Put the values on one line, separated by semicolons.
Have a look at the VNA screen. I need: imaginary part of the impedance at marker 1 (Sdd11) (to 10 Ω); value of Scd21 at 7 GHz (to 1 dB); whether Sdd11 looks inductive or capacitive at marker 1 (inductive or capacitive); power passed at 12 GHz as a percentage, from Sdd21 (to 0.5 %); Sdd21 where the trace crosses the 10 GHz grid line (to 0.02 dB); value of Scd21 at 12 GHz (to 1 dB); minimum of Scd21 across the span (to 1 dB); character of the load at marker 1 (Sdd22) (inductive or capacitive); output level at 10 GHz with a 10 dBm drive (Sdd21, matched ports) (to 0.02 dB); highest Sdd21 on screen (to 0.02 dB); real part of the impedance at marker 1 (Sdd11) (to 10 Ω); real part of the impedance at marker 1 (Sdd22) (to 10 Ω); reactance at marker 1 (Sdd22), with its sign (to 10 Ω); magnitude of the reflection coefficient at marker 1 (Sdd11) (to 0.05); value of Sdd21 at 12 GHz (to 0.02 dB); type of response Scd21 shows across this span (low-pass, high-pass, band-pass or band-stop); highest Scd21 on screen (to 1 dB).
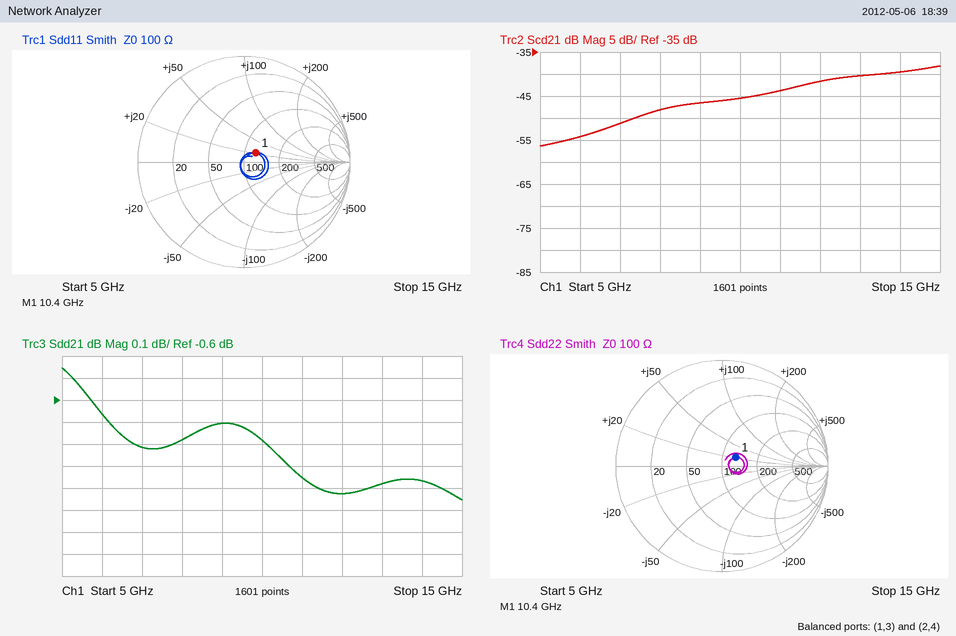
+20 Ω; -51 dB; inductive; 79.0 %; -0.78 dB; -42 dB; -56 dB; inductive; 9.22 dBm; -0.46 dB; 120 Ω; 130 Ω; +20 Ω; 0.15; -1.02 dB; high-pass; -38 dB
